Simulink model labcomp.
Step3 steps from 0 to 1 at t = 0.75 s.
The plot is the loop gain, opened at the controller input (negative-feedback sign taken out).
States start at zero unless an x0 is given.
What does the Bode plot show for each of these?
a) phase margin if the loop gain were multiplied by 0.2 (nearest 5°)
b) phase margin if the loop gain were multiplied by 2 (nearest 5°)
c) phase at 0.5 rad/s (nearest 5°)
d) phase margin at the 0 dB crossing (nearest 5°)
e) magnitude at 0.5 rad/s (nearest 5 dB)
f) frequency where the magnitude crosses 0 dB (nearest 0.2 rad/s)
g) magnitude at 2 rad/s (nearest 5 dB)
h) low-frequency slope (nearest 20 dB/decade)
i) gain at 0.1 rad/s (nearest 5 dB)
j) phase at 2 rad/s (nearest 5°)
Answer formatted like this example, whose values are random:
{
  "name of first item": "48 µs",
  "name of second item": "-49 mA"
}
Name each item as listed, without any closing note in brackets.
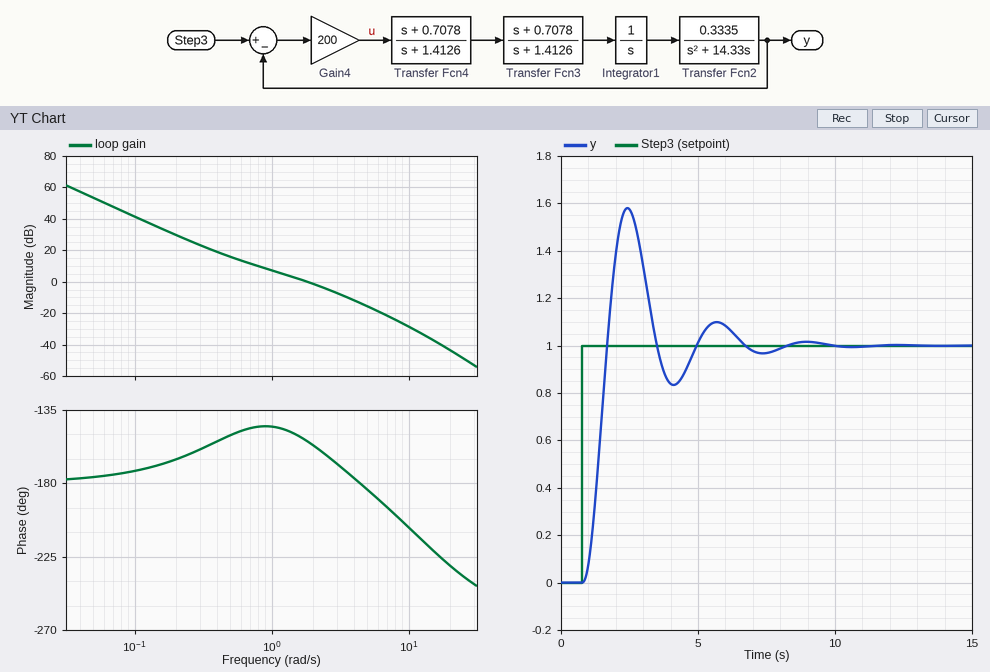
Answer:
{
  "phase margin if the loop gain were multiplied by 0.2": "30°",
  "phase margin if the loop gain were multiplied by 2": "15°",
  "phase at 0.5 rad/s": "-150°",
  "phase margin at the 0 dB crossing": "25°",
  "magnitude at 0.5 rad/s": "15 dB",
  "frequency where the magnitude crosses 0 dB": "1.8 rad/s",
  "magnitude at 2 rad/s": "0 dB",
  "low-frequency slope": "-40 dB/decade",
  "gain at 0.1 rad/s": "40 dB",
  "phase at 2 rad/s": "-155°"
}
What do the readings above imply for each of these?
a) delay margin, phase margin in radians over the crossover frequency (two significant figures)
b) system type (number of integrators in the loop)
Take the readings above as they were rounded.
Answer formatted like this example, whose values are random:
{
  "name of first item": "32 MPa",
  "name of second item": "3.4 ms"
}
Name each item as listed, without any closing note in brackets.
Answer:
{
  "delay margin, phase margin in radians over the crossover frequency": "0.24 s",
  "system type": "2"
}
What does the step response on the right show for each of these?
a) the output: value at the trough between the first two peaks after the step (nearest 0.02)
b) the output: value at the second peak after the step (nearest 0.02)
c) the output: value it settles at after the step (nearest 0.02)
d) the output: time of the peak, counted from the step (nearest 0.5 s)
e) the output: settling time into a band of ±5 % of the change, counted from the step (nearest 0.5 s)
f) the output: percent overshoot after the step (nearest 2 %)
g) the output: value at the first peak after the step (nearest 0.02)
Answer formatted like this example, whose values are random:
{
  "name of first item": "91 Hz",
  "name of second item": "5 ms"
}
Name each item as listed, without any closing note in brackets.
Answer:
{
  "the output: value at the trough between the first two peaks after the step": "0.84",
  "the output: value at the second peak after the step": "1.10",
  "the output: value it settles at after the step": "1.00",
  "the output: time of the peak, counted from the step": "1.5 s",
  "the output: settling time into a band of ±5 % of the change, counted from the step": "5.5 s",
  "the output: percent overshoot after the step": "58 %",
  "the output: value at the first peak after the step": "1.58"
}
